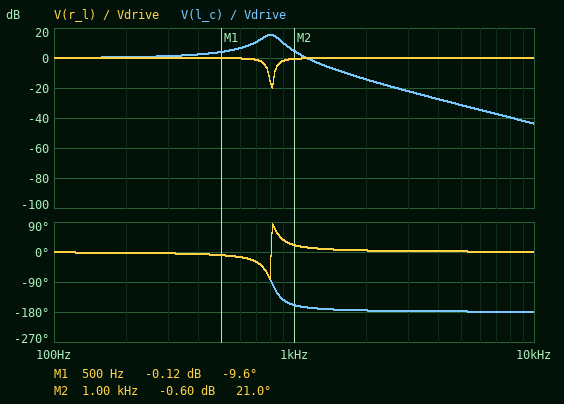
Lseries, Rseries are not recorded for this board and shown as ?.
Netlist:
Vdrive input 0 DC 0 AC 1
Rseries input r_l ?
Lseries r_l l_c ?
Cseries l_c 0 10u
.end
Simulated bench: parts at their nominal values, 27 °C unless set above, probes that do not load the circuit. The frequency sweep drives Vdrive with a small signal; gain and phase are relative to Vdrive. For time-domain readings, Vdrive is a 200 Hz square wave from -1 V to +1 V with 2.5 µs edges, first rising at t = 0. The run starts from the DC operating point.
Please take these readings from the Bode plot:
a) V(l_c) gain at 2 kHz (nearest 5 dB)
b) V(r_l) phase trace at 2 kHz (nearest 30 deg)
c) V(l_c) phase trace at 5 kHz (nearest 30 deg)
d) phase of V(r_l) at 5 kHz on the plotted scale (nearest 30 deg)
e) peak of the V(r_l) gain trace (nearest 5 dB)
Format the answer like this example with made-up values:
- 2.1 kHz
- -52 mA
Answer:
- -15 dB
- 0 deg
- -180 deg
- 0 deg
- 0 dB
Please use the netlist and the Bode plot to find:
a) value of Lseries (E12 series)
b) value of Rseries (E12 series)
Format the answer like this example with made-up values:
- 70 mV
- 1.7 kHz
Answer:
- 3.9 mH
- 3.3 Ω
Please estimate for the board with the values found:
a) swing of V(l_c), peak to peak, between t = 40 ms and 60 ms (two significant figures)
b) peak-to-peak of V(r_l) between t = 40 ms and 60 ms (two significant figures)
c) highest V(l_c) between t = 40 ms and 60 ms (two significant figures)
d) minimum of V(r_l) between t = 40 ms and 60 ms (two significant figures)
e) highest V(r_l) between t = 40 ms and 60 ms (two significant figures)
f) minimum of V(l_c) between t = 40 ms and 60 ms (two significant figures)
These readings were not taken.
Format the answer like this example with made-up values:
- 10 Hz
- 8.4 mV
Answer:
- 4.3 V
- 2.3 V
- 2.1 V
- -1.2 V
- 1.2 V
- -2.1 V
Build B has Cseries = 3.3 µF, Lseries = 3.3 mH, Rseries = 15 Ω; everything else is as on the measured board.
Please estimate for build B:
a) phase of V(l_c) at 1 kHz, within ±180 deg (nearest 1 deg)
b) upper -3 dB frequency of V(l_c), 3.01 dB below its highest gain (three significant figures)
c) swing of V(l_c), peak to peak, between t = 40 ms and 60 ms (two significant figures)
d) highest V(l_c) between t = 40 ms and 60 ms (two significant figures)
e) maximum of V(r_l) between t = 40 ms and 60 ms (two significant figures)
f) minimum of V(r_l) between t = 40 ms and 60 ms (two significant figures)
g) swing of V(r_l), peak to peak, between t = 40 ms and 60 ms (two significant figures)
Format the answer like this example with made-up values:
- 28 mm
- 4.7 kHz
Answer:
- -29 deg
- 1.77 kHz
- 3.9 V
- 1.9 V
- 1.3 V
- -1.3 V
- 2.6 V
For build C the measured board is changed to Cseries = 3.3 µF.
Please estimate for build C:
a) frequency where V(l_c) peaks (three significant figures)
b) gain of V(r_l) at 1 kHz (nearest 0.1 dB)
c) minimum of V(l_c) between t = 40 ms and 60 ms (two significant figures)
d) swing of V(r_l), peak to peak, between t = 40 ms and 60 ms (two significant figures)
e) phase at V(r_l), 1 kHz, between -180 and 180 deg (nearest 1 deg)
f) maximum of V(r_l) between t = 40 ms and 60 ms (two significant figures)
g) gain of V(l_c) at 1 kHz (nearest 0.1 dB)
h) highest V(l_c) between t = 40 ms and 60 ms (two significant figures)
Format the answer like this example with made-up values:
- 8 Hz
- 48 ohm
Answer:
- 1.40 kHz
- -0.1 dB
- -3.6 V
- 2.5 V
- -8 deg
- 1.2 V
- 6.1 dB
- 3.6 V
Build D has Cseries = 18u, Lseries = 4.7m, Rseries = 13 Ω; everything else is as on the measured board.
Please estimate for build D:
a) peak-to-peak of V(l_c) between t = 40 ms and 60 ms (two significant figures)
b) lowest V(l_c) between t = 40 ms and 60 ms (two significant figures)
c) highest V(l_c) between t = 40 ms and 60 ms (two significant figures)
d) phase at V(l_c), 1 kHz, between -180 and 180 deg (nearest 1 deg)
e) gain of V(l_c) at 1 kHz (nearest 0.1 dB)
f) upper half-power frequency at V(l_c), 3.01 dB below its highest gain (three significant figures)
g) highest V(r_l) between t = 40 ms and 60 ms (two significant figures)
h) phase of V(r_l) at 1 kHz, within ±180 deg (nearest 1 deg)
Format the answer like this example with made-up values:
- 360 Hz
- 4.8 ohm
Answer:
- 3.0 V
- -1.5 V
- 1.5 V
- -148 deg
- -8.8 dB
- 650 Hz
- 1.2 V
- 32 deg
